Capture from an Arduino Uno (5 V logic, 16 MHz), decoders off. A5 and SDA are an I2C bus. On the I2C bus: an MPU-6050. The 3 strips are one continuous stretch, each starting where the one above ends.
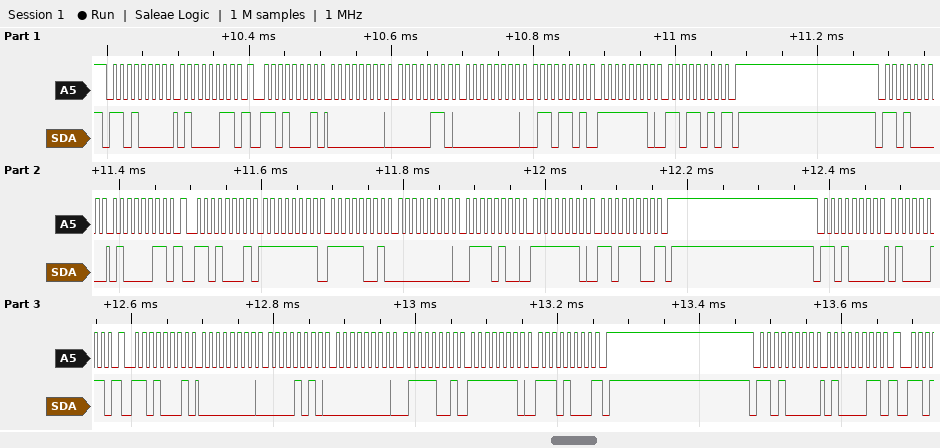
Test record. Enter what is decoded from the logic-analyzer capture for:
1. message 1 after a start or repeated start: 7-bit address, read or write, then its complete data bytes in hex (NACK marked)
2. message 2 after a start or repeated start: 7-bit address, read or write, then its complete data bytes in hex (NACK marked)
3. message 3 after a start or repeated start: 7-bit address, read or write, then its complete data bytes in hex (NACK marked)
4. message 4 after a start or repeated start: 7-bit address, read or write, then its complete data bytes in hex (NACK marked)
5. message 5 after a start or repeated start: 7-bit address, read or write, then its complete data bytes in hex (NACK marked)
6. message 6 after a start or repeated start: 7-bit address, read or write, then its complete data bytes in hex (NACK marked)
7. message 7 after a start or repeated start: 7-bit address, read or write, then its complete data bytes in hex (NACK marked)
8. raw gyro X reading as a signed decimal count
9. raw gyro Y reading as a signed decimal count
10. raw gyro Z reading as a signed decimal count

0x68 write: 43
0x68 read: 00 06 00 6D FE DA NACK
0x68 write: 43
0x68 read: FF F9 00 74 FE DC NACK
0x68 write: 43
0x68 read: 00 0A 00 79 FE E8 NACK
0x68 write: 43
6
109
-294
